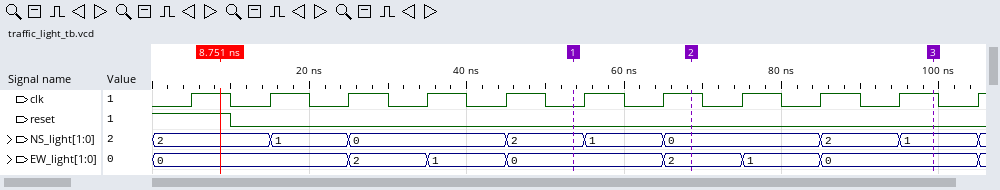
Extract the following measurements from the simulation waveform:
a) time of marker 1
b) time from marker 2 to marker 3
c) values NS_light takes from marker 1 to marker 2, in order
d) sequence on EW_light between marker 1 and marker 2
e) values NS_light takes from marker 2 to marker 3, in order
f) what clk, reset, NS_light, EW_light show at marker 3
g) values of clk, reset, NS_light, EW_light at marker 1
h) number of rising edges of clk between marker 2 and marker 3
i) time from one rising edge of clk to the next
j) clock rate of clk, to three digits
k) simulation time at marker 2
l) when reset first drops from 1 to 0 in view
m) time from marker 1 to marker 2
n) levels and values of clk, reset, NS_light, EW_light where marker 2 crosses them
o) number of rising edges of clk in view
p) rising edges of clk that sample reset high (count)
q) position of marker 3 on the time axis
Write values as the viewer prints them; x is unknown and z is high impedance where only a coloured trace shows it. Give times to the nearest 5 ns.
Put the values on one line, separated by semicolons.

55 ns; 30 ns; 2, 1, 0; 0, 2; 0, 2, 1; clk=1, reset=0, NS_light=1, EW_light=0; clk=0, reset=0, NS_light=2, EW_light=0; 3; 10 ns; 100 MHz; 70 ns; 10 ns; 15 ns; clk=1, reset=0, NS_light=0, EW_light=2; 11; 1; 100 ns
